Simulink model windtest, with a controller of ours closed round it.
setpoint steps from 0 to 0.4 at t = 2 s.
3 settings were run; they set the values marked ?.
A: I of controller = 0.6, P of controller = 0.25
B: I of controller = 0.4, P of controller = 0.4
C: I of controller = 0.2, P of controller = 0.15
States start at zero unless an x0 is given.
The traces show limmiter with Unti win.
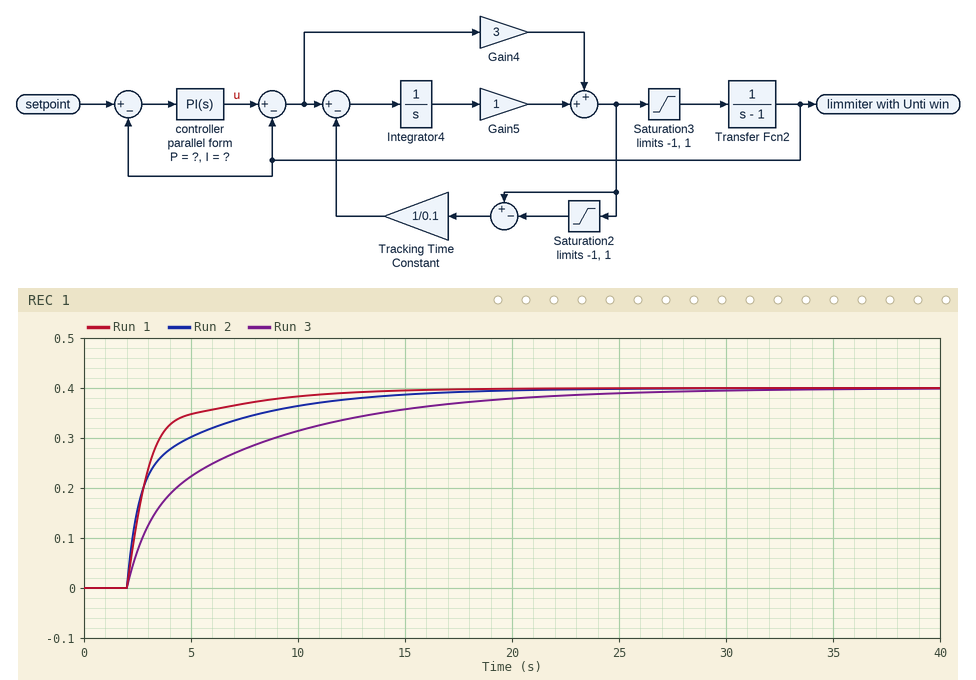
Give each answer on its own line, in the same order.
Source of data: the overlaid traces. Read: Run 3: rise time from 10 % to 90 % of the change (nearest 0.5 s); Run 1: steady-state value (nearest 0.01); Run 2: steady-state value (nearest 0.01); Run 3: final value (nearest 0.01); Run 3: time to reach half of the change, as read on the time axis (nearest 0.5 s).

13.0 s
0.40
0.40
0.40
4.5 s
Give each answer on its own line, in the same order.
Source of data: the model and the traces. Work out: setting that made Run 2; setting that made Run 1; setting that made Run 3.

B
A
C
